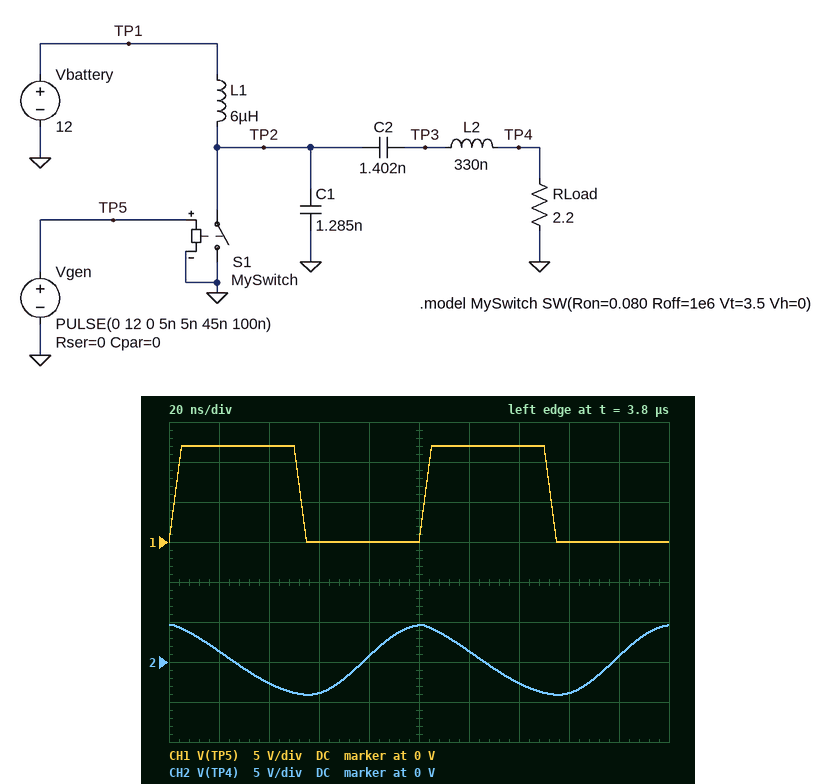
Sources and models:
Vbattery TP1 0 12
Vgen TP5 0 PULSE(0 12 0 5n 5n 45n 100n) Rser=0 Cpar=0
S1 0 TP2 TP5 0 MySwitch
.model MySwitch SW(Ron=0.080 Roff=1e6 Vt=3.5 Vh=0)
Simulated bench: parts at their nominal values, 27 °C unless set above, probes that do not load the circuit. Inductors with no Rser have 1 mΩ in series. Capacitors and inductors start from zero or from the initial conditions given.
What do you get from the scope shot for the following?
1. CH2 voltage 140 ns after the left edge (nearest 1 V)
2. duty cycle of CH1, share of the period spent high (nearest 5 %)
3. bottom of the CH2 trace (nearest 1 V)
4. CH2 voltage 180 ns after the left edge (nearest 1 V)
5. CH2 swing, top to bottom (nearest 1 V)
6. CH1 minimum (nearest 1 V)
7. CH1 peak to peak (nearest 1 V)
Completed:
-3 V
50 %
-4 V
1 V
9 V
0 V
12 V
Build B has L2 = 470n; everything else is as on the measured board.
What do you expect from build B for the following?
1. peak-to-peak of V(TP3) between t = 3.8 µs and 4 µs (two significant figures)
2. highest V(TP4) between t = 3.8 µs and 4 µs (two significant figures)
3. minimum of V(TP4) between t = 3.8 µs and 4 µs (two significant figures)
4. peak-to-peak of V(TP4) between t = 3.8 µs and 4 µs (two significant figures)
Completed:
57 V
2.7 V
-2.2 V
4.8 V
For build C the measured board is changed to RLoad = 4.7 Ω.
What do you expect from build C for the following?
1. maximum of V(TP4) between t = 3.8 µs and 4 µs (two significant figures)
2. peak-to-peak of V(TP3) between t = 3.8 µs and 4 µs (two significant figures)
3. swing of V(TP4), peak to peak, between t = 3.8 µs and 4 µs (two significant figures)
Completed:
9.0 V
71 V
17 V
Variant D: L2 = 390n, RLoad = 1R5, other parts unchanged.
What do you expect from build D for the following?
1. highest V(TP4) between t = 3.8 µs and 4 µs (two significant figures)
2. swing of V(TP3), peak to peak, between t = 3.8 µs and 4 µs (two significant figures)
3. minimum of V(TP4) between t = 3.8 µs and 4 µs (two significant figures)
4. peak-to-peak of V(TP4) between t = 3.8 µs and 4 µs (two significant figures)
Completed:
2.4 V
65 V
-2.1 V
4.5 V
